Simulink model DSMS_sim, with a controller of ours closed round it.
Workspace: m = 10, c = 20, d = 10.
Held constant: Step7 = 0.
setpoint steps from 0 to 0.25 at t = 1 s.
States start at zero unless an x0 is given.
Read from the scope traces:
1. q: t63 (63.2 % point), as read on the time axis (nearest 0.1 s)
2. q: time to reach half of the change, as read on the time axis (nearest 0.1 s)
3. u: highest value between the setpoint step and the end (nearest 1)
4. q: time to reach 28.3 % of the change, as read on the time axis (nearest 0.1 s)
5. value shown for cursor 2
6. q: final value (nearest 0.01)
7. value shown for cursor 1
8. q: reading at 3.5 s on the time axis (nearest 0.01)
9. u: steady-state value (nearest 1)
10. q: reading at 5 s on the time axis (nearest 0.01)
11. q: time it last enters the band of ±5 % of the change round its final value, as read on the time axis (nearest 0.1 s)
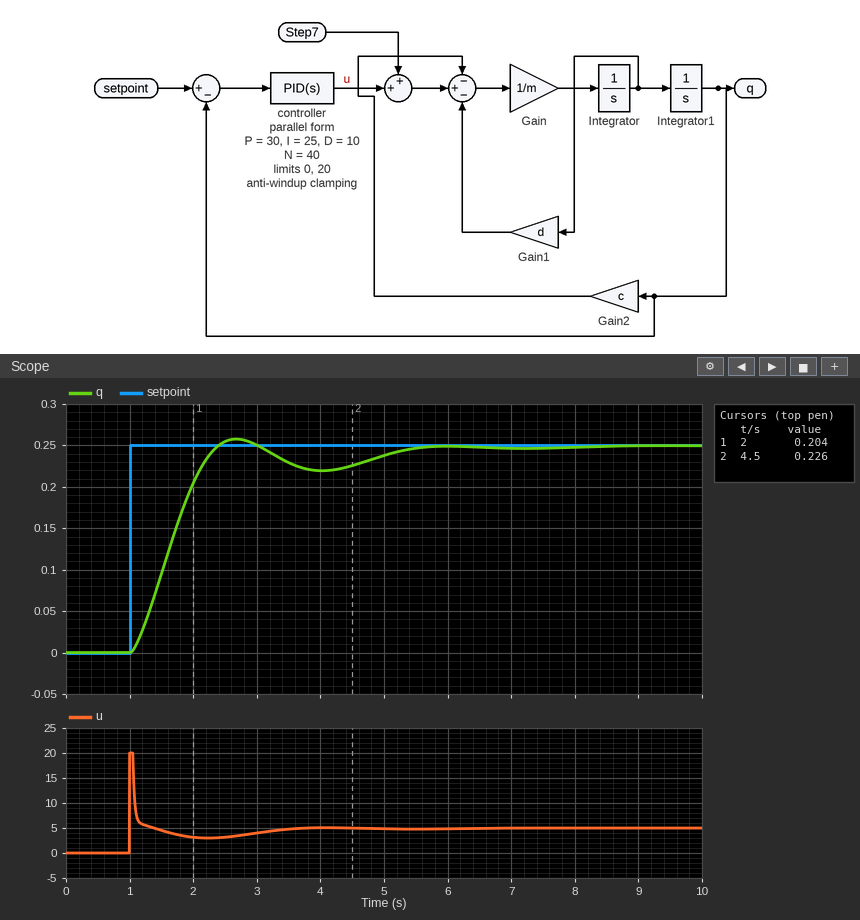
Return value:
1.8 s
1.6 s
20
1.4 s
0.226
0.25
0.204
0.23
5
0.24
5.0 s
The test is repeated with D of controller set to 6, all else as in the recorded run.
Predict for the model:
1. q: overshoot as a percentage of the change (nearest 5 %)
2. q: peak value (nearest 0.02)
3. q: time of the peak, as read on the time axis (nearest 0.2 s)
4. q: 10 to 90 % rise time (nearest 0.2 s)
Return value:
10 %
0.28
2.6 s
0.8 s
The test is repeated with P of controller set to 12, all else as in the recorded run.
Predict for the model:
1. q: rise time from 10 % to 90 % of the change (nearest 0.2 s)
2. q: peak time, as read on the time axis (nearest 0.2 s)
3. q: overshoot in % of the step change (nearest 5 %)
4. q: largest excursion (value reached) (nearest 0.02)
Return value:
1.4 s
3.6 s
10 %
0.28
